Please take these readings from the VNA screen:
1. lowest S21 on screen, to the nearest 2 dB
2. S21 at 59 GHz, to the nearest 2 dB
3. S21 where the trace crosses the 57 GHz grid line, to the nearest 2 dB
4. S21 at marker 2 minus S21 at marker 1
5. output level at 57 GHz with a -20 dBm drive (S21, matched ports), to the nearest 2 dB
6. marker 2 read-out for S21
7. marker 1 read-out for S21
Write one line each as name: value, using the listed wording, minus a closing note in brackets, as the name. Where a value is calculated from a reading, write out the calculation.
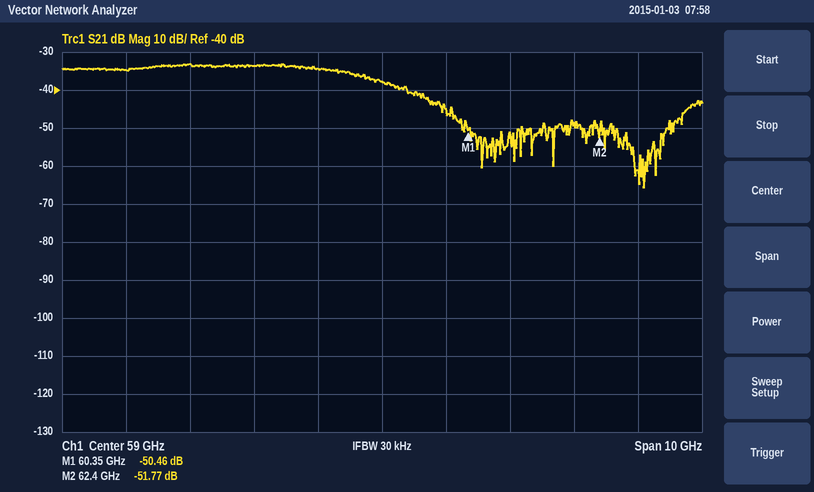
lowest S21 on screen, to the nearest 2 dB: -66 dB
S21 at 59 GHz, to the nearest 2 dB: -38 dB
S21 where the trace crosses the 57 GHz grid line, to the nearest 2 dB: -34 dB
S21 at marker 2 minus S21 at marker 1: -51.77 − (-50.46) = -1.31 dB
output level at 57 GHz with a -20 dBm drive (S21, matched ports), to the nearest 2 dB: -20 dBm + (-34 dB) = -54 dBm
marker 2 read-out for S21: -51.77 dB
marker 1 read-out for S21: -50.46 dB
